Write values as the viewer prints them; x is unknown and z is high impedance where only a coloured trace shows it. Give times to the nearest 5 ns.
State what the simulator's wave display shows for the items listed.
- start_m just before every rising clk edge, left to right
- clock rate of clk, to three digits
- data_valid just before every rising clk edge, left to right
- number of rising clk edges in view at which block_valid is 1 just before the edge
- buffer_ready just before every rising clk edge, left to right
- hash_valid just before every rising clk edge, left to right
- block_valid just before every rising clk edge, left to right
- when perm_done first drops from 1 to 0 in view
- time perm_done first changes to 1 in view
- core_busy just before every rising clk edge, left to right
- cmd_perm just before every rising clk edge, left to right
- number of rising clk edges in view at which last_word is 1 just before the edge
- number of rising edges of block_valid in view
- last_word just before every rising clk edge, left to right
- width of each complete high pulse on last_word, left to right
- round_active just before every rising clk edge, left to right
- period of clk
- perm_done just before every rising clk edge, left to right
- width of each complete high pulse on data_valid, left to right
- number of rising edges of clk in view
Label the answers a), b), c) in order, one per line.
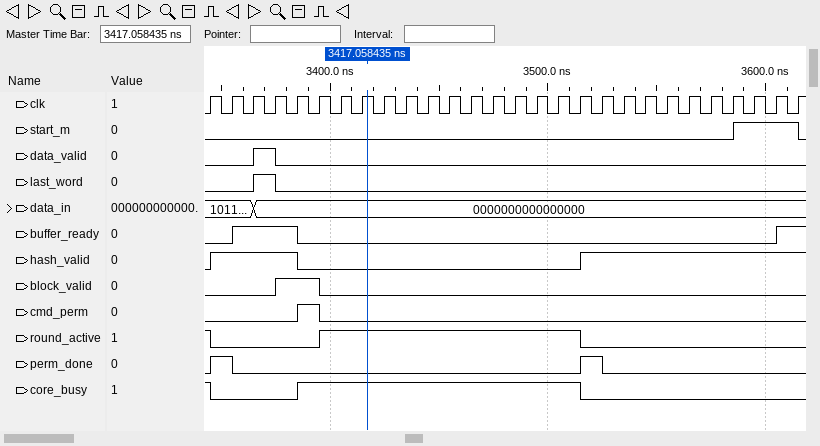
a) 0 0 0 0 0 0 0 0 0 0 0 0 0 0 0 0 0 0 0 0 0 0 0 0 0 1 1 1
b) 100 MHz
c) 0 0 0 1 0 0 0 0 0 0 0 0 0 0 0 0 0 0 0 0 0 0 0 0 0 0 0 0
d) 2
e) 0 0 1 1 1 0 0 0 0 0 0 0 0 0 0 0 0 0 0 0 0 0 0 0 0 0 0 1
f) 0 1 1 1 1 0 0 0 0 0 0 0 0 0 0 0 0 0 1 1 1 1 1 1 1 1 1 1
g) 0 0 0 0 1 1 0 0 0 0 0 0 0 0 0 0 0 0 0 0 0 0 0 0 0 0 0 0
h) 3355 ns
i) 3345 ns
j) 1 0 0 0 0 1 1 1 1 1 1 1 1 1 1 1 1 1 0 0 0 0 0 0 0 0 0 0
k) 0 0 0 0 0 1 0 0 0 0 0 0 0 0 0 0 0 0 0 0 0 0 0 0 0 0 0 0
l) 1
m) 1
n) 0 0 0 1 0 0 0 0 0 0 0 0 0 0 0 0 0 0 0 0 0 0 0 0 0 0 0 0
o) 10 ns
p) 1 0 0 0 0 0 1 1 1 1 1 1 1 1 1 1 1 1 0 0 0 0 0 0 0 0 0 0
q) 10 ns
r) 0 1 0 0 0 0 0 0 0 0 0 0 0 0 0 0 0 0 1 0 0 0 0 0 0 0 0 0
s) 10 ns
t) 28
